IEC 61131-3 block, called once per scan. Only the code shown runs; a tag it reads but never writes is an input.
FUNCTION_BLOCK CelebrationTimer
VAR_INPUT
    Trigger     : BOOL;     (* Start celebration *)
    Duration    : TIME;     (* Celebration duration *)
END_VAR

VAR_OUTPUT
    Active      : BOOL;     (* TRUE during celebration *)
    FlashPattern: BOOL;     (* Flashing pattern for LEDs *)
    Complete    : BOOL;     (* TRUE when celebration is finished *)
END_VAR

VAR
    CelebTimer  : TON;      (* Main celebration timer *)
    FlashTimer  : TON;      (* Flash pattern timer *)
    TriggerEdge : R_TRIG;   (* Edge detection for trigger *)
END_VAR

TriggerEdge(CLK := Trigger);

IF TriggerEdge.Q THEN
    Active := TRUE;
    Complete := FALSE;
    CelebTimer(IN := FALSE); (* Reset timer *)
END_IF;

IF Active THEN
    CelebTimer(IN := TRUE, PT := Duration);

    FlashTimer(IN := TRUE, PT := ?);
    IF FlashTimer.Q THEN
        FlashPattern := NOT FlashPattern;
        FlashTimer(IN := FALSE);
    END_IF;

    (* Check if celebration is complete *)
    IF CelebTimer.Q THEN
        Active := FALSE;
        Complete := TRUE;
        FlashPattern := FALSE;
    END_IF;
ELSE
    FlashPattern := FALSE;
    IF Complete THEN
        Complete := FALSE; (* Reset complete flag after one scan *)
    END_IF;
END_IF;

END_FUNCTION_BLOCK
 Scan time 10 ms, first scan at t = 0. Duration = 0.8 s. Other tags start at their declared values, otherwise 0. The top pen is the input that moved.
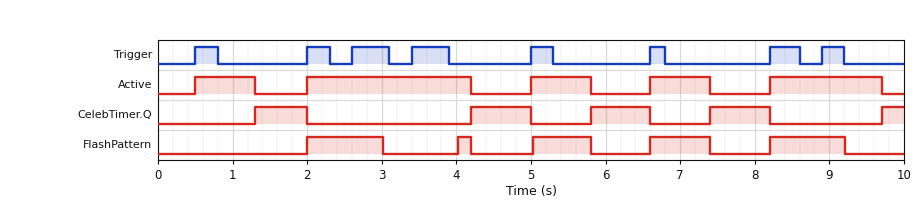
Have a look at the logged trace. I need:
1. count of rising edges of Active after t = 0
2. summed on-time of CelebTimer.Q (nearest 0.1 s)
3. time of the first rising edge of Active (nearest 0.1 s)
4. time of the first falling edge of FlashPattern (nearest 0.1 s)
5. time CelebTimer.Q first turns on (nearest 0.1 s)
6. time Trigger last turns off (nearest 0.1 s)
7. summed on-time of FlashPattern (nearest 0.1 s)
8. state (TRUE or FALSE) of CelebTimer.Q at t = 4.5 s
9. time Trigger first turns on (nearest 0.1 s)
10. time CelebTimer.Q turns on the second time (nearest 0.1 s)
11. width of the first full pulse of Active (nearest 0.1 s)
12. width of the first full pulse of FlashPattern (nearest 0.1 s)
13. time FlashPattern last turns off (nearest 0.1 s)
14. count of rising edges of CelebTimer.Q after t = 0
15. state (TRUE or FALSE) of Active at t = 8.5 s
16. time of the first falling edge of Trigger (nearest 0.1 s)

5
3.4 s
0.5 s
3.0 s
1.3 s
9.2 s
3.8 s
TRUE
0.5 s
4.2 s
0.8 s
1.0 s
9.2 s
5
TRUE
0.8 s
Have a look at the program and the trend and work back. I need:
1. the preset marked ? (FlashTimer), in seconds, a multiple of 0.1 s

1.0 s
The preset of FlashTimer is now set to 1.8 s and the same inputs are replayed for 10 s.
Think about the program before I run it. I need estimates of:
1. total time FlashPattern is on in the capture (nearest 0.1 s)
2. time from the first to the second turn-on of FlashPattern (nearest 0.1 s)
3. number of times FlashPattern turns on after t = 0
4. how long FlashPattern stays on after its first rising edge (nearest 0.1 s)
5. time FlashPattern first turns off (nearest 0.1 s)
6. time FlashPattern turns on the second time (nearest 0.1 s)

3.9 s
4.3 s
3
1.8 s
4.1 s
6.6 s
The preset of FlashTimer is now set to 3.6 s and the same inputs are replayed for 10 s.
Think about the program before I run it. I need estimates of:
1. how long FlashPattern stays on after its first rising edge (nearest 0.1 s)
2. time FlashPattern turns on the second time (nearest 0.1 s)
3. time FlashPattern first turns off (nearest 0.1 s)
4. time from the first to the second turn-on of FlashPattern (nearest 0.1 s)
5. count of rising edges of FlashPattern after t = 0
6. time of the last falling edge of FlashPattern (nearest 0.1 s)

0.1 s
8.2 s
4.2 s
4.1 s
2
9.7 s
